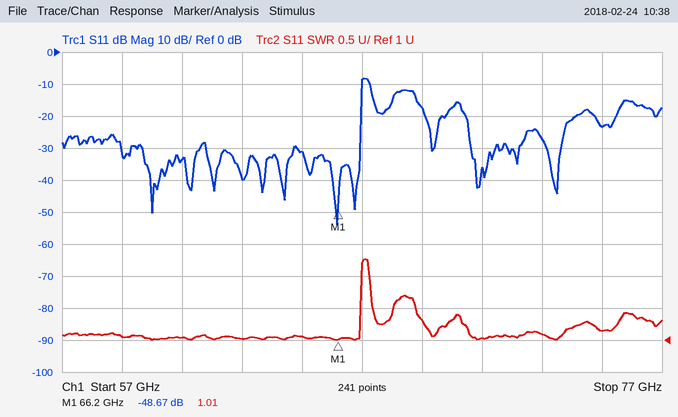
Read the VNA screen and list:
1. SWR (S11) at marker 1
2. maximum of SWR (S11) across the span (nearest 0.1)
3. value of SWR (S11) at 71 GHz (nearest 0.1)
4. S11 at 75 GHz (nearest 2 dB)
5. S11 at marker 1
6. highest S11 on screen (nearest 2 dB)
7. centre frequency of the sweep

1.01
2.3
1.0
-24 dB
-48.67 dB
-8 dB
67 GHz
